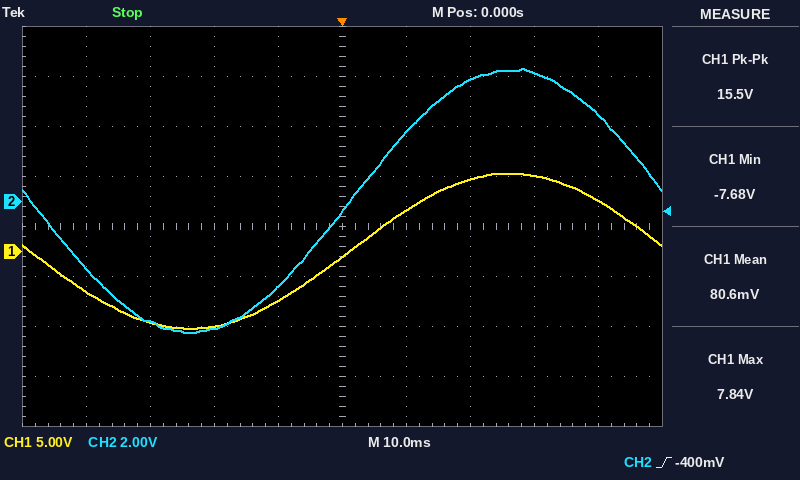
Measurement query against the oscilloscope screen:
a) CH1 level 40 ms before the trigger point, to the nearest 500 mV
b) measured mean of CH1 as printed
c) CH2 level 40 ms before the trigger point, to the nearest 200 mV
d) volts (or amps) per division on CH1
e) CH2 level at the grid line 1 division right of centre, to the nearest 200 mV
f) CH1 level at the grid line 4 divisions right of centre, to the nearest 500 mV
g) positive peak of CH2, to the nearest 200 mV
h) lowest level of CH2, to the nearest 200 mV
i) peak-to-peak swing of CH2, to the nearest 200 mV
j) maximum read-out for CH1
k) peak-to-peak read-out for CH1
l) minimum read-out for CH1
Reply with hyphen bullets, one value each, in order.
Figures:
- -4.0 V
- 80.6 mV
- -2.6 V
- 5 V
- 2.8 V
- 5.0 V
- 5.4 V
- -5.2 V
- 10.6 V
- 7.84 V
- 15.5 V
- -7.68 V
